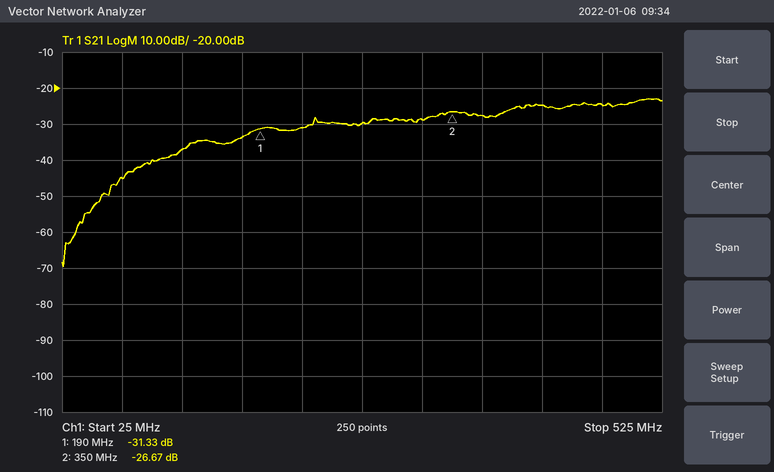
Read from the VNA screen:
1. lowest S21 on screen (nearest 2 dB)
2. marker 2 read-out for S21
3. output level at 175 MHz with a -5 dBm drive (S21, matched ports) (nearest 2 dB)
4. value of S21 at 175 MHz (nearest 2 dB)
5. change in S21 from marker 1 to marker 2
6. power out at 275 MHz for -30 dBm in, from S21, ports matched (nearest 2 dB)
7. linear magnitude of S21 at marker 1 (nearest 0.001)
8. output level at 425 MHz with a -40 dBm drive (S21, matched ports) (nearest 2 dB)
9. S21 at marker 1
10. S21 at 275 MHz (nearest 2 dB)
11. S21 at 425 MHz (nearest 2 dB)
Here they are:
-70 dB
-26.67 dB
-38 dBm
-34 dB
4.66 dB
-60 dBm
0.027
-64 dBm
-31.33 dB
-30 dB
-24 dB
